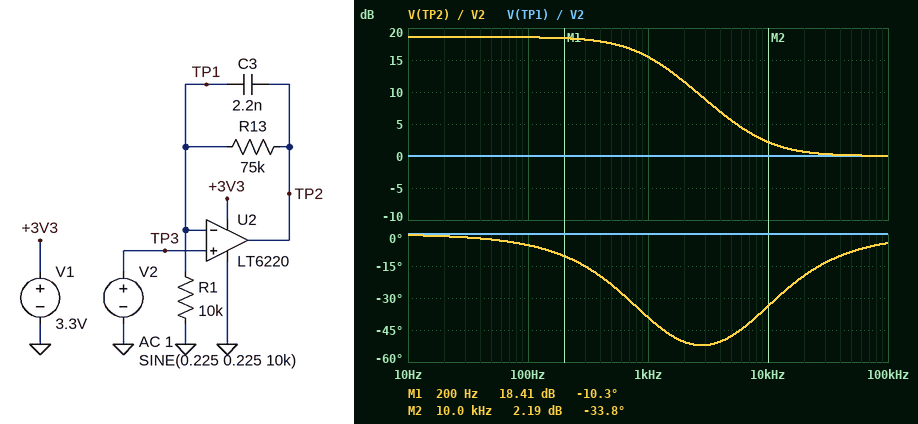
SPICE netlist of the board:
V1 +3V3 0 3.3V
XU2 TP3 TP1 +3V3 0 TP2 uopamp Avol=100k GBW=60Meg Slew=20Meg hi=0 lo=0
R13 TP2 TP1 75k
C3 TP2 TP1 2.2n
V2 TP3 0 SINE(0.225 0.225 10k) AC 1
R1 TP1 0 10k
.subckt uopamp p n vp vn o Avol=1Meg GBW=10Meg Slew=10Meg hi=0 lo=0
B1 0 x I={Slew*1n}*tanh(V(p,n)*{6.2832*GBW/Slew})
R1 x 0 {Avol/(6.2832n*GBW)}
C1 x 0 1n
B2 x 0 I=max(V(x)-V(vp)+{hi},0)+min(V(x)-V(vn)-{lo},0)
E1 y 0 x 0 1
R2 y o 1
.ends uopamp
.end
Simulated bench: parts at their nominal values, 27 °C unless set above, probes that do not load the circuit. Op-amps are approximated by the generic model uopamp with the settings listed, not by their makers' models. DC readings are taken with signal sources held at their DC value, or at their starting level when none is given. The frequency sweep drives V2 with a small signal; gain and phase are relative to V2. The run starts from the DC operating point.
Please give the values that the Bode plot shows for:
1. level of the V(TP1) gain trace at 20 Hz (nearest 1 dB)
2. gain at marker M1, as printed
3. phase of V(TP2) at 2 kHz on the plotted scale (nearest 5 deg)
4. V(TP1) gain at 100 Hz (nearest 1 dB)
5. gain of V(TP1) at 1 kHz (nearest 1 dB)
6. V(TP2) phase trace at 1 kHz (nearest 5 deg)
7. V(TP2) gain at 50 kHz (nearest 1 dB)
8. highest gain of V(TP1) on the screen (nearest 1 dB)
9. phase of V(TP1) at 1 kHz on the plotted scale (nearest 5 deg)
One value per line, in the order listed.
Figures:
0 dB
18.41 dB
-50 deg
0 dB
0 dB
-40 deg
0 dB
0 dB
0 deg
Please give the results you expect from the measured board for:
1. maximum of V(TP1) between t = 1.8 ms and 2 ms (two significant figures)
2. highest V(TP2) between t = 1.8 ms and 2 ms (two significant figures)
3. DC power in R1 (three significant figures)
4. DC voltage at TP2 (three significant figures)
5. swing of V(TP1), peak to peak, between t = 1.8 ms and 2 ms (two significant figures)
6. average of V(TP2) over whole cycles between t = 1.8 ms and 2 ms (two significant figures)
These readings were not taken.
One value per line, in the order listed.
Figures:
450 mV
2.2 V
5.06 µW
1.91 V
450 mV
1.9 V
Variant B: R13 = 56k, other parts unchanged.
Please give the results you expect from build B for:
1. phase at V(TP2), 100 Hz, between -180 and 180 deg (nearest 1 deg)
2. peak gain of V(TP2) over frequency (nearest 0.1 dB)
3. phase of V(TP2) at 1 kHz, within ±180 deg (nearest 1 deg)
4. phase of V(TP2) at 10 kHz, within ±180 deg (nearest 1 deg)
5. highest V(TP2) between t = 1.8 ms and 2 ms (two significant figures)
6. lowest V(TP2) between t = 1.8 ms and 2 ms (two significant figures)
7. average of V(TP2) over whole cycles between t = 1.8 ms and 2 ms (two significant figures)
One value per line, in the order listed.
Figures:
-4 deg
16.4 dB
-31 deg
-33 deg
1.8 V
1.2 V
1.5 V
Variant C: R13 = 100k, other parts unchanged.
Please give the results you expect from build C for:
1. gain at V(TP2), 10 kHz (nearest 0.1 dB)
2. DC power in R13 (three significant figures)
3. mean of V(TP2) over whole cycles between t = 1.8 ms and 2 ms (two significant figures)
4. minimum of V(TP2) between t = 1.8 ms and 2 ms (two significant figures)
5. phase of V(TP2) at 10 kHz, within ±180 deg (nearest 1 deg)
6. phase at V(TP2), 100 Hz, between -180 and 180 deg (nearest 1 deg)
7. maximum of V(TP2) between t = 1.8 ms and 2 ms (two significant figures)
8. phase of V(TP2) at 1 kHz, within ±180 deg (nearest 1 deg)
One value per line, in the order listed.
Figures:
2.1 dB
50.6 µW
2.5 V
2.2 V
-34 deg
-7 deg
2.8 V
-47 deg
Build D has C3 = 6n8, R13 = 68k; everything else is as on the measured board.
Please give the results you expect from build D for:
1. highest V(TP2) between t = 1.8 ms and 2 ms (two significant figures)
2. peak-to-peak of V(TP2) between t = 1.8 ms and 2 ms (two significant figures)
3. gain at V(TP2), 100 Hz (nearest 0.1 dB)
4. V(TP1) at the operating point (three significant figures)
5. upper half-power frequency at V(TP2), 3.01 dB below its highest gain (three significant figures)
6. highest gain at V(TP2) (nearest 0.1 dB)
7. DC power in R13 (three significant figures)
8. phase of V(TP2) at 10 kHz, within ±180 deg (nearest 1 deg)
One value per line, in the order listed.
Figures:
2.0 V
470 mV
17.5 dB
225 mV
350 Hz
17.8 dB
34.4 µW
-13 deg
